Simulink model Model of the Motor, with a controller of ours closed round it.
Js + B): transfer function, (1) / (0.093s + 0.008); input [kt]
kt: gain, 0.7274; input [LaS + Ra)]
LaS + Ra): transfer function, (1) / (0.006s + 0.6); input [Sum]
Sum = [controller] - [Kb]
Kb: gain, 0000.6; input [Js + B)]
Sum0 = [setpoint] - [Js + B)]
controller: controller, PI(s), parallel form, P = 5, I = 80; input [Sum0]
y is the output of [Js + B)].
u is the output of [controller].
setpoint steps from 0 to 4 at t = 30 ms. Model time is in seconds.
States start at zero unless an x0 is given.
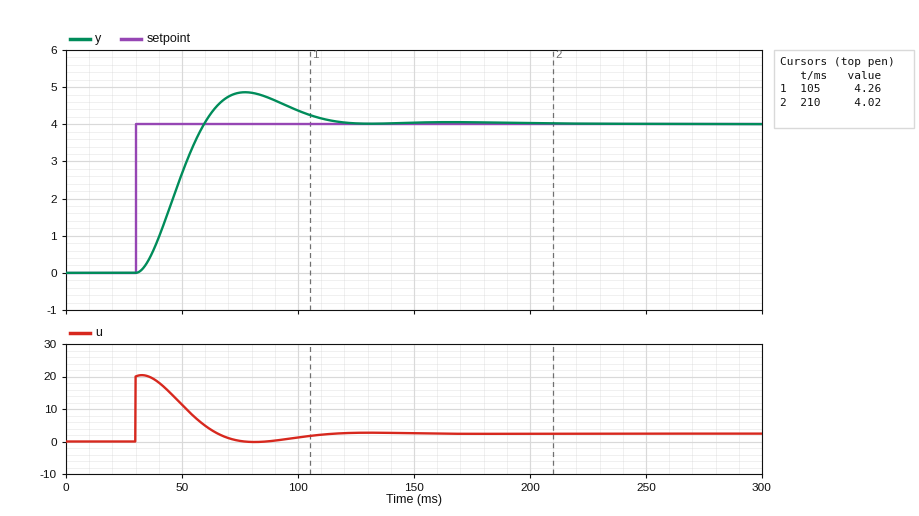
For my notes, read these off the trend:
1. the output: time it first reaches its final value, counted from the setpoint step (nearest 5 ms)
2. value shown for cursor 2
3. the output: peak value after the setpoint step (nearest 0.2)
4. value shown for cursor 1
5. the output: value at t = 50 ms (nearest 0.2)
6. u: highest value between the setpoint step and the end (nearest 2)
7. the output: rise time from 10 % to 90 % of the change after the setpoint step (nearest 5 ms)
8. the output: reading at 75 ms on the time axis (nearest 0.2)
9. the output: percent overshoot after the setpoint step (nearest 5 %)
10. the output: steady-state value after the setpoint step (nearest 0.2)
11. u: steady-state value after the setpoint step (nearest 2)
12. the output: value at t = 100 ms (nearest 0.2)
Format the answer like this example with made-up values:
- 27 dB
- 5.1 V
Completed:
- 30 ms
- 4.02
- 4.8
- 4.26
- 2.6
- 20
- 20 ms
- 4.8
- 20 %
- 4.0
- 2
- 4.4
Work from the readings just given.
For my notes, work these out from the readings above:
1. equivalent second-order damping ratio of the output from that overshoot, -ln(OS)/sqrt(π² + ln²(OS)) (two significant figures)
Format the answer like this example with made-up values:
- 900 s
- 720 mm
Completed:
- 0.46
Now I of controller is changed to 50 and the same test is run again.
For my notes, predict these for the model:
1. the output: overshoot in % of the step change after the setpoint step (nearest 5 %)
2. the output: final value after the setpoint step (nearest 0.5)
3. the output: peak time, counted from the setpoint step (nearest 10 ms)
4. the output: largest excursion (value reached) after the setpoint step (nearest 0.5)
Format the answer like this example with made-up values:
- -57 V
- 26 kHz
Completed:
- 15 %
- 4.0
- 50 ms
- 4.5
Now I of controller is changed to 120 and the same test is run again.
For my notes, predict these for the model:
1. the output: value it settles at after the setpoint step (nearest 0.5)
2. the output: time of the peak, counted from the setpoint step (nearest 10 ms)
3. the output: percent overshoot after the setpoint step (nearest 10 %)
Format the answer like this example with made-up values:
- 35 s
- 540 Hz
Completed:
- 4.0
- 50 ms
- 30 %
